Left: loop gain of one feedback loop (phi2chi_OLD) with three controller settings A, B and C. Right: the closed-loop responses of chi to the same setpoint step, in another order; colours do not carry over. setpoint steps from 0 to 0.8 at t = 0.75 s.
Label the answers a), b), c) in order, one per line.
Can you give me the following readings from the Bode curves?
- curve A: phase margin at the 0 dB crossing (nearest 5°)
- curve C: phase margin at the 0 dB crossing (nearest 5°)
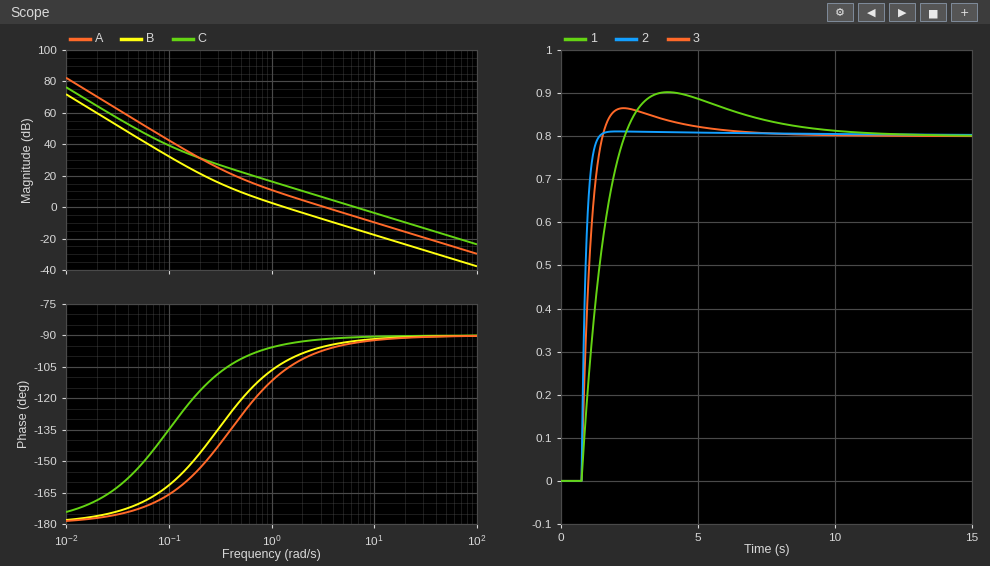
a) 85°
b) 90°
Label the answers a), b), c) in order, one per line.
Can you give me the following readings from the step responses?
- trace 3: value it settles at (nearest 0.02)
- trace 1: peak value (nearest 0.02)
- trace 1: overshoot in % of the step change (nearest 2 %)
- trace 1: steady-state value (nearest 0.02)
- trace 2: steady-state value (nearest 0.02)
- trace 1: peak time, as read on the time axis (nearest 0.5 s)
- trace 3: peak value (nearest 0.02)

a) 0.80
b) 0.90
c) 12 %
d) 0.80
e) 0.80
f) 4.0 s
g) 0.86
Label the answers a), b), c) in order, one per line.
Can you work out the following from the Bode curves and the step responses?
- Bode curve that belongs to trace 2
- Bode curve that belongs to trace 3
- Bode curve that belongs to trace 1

a) C
b) A
c) B
